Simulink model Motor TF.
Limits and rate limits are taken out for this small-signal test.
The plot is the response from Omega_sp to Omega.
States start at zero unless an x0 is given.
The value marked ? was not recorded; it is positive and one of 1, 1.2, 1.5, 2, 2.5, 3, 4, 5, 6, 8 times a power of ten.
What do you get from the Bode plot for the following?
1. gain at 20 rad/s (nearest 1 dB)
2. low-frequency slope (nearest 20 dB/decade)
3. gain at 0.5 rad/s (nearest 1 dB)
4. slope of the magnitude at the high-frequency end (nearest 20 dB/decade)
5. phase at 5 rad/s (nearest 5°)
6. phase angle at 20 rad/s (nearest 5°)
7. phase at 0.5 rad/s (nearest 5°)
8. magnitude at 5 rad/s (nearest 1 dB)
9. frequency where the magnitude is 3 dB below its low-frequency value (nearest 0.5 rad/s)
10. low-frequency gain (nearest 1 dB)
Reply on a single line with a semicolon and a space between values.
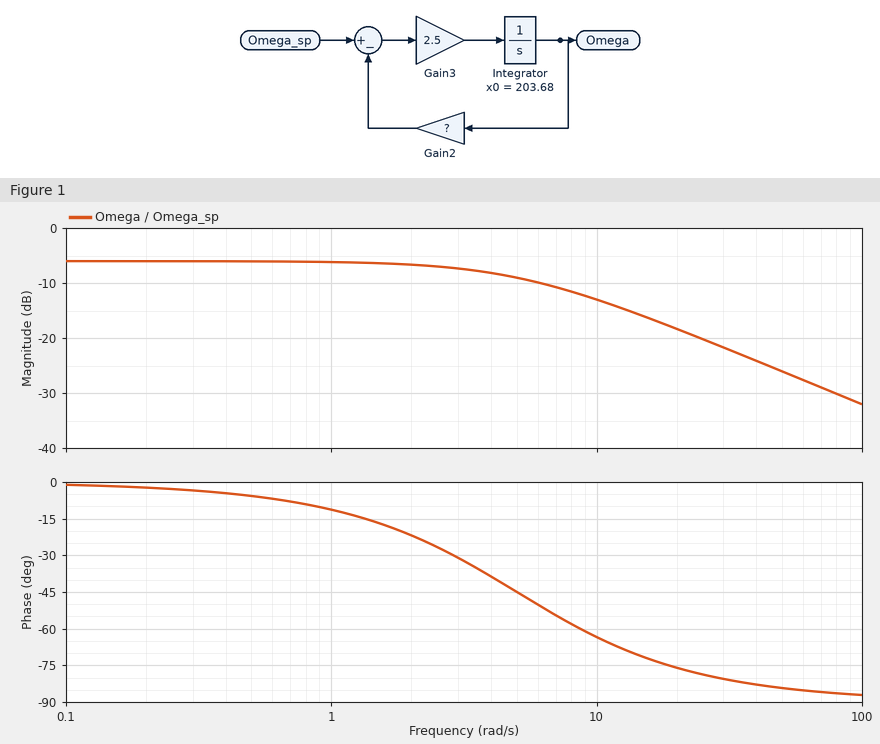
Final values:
-18 dB; 0 dB/decade; -6 dB; -20 dB/decade; -45°; -75°; -5°; -9 dB; 5.0 rad/s; -6 dB
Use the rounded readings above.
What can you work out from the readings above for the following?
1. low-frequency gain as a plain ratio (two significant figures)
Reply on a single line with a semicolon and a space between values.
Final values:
0.50
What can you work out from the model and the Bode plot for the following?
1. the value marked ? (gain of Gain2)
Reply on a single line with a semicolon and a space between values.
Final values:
2
